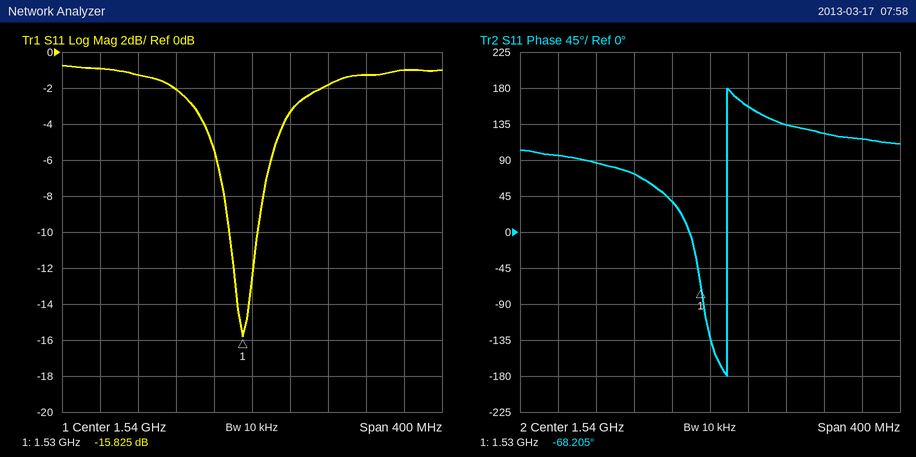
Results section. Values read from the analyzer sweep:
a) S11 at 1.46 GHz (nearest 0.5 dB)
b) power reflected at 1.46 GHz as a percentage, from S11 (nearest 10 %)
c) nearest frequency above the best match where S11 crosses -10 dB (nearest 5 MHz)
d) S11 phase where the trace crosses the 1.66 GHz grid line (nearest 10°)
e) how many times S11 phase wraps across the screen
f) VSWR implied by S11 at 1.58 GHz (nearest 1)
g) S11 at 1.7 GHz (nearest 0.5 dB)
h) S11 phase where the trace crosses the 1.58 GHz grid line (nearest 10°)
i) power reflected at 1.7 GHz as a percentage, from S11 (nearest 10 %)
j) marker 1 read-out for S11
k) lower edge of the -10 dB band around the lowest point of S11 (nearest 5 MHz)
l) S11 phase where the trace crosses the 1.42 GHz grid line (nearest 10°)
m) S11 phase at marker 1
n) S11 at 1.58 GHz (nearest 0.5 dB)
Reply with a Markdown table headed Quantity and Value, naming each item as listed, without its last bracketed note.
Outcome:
| Quantity | Value |
|---|---|
| S11 at 1.46 GHz | -2.0 dB |
| power reflected at 1.46 GHz as a percentage, from S11 | 60 % |
| nearest frequency above the best match where S11 crosses -10 dB | 1.545 GHz |
| S11 phase where the trace crosses the 1.66 GHz grid line | 120° |
| how many times S11 phase wraps across the screen | 1 |
| VSWR implied by S11 at 1.58 GHz | 5 |
| S11 at 1.7 GHz | -1.0 dB |
| S11 phase where the trace crosses the 1.58 GHz grid line | 160° |
| power reflected at 1.7 GHz as a percentage, from S11 | 80 % |
| marker 1 read-out for S11 | -15.825 dB |
| lower edge of the -10 dB band around the lowest point of S11 | 1.515 GHz |
| S11 phase where the trace crosses the 1.42 GHz grid line | 90° |
| S11 phase at marker 1 | -68.205° |
| S11 at 1.58 GHz | -3.5 dB |
